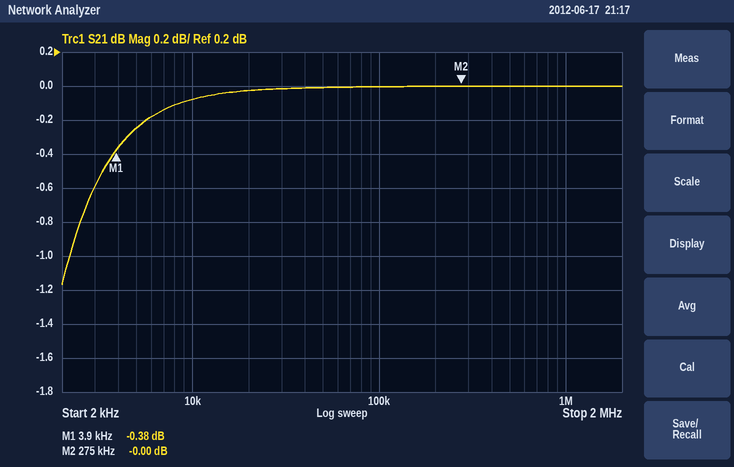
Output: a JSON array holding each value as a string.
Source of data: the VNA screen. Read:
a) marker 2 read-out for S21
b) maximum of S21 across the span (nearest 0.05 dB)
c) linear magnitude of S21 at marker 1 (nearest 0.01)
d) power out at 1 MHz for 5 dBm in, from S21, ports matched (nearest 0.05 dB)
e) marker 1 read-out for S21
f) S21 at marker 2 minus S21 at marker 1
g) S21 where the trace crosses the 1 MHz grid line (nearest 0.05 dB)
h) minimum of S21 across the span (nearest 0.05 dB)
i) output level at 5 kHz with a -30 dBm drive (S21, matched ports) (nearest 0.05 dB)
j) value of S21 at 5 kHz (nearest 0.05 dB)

["-0.00 dB", "0.00 dB", "0.96", "5.00 dBm", "-0.38 dB", "0.38 dB", "0.00 dB", "-1.15 dB", "-30.25 dBm", "-0.25 dB"]
